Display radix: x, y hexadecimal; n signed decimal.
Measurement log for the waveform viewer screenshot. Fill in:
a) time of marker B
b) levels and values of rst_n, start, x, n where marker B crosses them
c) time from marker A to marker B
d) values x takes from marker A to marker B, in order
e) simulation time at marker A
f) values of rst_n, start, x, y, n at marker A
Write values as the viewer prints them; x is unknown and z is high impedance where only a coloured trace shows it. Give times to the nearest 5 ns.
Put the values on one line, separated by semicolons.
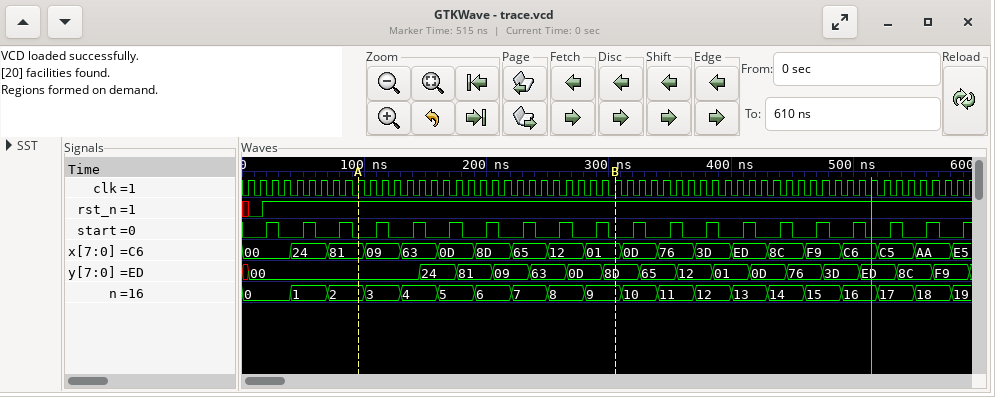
305 ns; rst_n=1, start=0, x=01, n=9; 210 ns; 81, 09, 63, 0D, 8D, 65, 12, 01; 95 ns; rst_n=1, start=0, x=81, y=00, n=2
